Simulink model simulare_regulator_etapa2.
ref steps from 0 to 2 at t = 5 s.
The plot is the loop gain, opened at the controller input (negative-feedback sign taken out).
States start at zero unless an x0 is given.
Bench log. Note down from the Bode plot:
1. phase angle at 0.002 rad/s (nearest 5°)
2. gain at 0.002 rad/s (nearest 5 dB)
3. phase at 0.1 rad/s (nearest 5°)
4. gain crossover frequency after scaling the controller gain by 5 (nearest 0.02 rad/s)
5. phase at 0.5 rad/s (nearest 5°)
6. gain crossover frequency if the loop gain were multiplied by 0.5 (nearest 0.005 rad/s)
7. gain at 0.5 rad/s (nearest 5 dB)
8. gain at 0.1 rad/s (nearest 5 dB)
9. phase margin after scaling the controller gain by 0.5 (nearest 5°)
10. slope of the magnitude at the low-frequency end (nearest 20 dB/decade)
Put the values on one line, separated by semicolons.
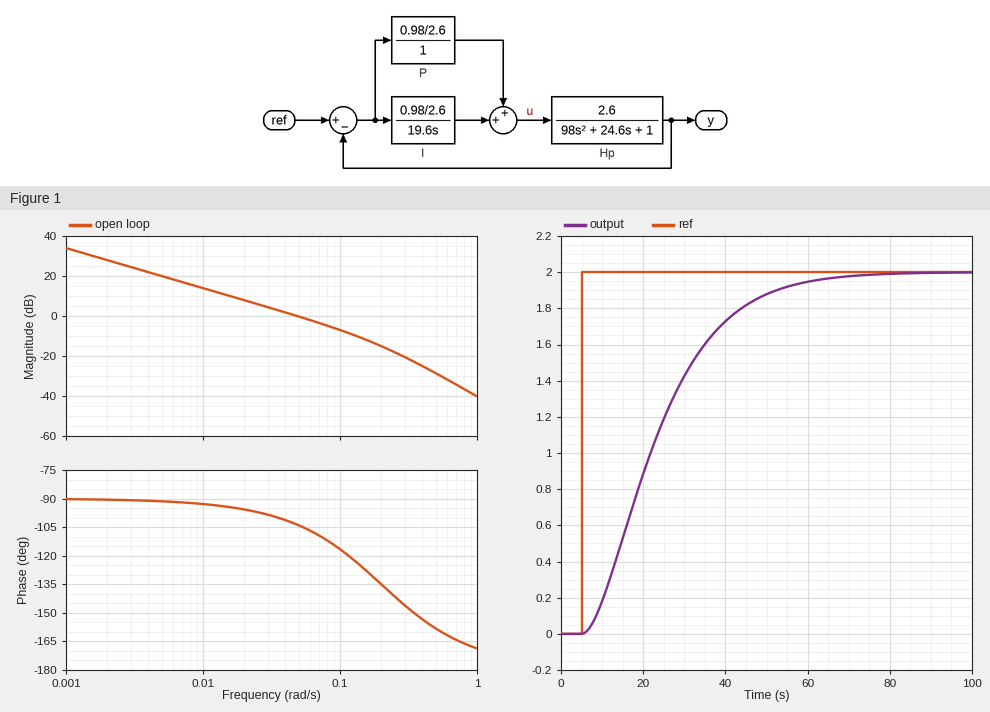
-90°; 30 dB; -115°; 0.18 rad/s; -160°; 0.025 rad/s; -30 dB; -5 dB; 85°; -20 dB/decade
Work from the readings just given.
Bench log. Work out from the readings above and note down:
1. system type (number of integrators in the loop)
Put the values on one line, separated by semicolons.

1
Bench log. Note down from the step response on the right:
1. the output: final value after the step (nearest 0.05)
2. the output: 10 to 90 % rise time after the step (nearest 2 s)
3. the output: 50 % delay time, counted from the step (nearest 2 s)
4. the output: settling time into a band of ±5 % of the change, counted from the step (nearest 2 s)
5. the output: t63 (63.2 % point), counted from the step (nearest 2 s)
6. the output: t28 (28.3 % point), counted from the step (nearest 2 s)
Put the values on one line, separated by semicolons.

2.00; 34 s; 16 s; 48 s; 22 s; 10 s
